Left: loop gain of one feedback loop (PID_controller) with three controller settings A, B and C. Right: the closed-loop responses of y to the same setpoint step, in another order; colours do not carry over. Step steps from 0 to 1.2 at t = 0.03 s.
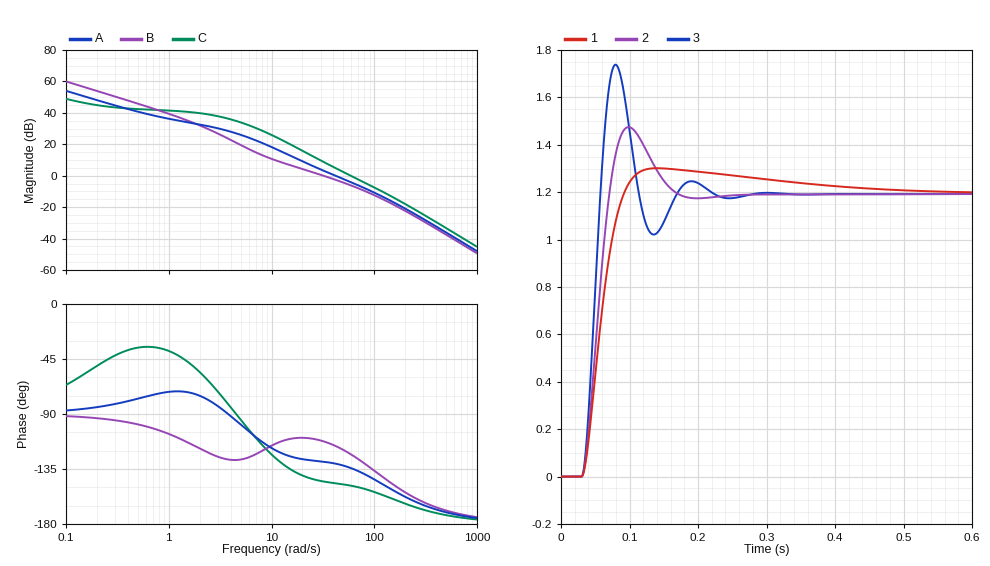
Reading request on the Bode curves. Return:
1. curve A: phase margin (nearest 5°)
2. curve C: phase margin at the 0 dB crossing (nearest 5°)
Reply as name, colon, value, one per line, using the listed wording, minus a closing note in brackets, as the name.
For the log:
curve A: phase margin: 50°
curve C: phase margin at the 0 dB crossing: 30°
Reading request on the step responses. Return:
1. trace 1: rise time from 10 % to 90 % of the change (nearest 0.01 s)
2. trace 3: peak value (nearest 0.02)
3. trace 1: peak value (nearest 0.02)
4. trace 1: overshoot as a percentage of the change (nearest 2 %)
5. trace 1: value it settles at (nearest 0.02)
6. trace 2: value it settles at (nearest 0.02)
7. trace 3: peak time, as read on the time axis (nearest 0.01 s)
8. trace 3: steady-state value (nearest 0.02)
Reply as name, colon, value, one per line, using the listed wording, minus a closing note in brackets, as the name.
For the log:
trace 1: rise time from 10 % to 90 % of the change: 0.04 s
trace 3: peak value: 1.74
trace 1: peak value: 1.30
trace 1: overshoot as a percentage of the change: 8 %
trace 1: value it settles at: 1.20
trace 2: value it settles at: 1.20
trace 3: peak time, as read on the time axis: 0.08 s
trace 3: steady-state value: 1.20
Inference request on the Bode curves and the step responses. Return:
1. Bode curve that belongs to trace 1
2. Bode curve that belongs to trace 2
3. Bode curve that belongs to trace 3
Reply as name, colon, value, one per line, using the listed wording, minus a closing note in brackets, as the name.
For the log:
Bode curve that belongs to trace 1: B
Bode curve that belongs to trace 2: A
Bode curve that belongs to trace 3: C
